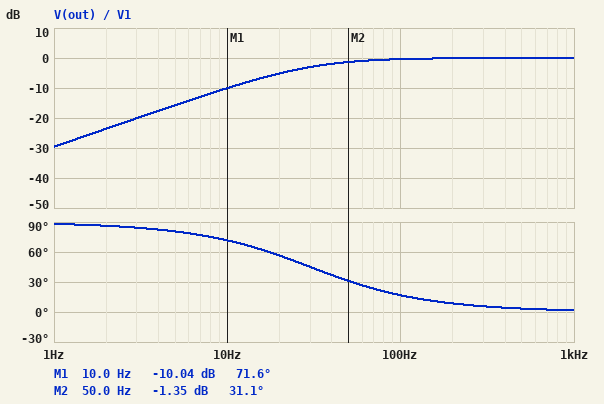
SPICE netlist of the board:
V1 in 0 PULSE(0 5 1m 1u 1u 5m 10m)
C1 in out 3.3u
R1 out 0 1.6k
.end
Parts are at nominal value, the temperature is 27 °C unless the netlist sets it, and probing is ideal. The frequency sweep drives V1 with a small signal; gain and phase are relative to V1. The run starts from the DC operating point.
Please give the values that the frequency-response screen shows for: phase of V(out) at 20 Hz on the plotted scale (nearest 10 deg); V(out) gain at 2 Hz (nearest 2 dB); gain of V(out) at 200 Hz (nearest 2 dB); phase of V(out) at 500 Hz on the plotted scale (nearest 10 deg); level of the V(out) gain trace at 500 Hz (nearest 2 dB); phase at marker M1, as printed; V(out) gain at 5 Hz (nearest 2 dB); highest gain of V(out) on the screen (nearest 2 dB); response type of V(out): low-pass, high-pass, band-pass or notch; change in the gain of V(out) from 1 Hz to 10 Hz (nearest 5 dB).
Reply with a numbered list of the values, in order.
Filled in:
1. 60 deg
2. -24 dB
3. 0 dB
4. 0 deg
5. 0 dB
6. 71.6 deg
7. -16 dB
8. 0 dB
9. high-pass
10. 20 dB
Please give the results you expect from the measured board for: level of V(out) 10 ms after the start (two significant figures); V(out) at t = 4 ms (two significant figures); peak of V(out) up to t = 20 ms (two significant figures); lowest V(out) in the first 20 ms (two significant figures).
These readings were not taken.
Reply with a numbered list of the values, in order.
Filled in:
1. -1.4 V
2. 2.8 V
3. 5.0 V
4. -3.5 V
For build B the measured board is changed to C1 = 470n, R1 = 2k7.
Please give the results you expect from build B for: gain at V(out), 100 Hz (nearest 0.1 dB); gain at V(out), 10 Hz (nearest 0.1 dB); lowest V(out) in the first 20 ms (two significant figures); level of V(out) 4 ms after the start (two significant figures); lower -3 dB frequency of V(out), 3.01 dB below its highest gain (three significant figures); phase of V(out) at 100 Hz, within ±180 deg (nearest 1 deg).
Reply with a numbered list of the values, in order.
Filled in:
1. -4.1 dB
2. -22.0 dB
3. -4.9 V
4. 470 mV
5. 125 Hz
6. 51 deg
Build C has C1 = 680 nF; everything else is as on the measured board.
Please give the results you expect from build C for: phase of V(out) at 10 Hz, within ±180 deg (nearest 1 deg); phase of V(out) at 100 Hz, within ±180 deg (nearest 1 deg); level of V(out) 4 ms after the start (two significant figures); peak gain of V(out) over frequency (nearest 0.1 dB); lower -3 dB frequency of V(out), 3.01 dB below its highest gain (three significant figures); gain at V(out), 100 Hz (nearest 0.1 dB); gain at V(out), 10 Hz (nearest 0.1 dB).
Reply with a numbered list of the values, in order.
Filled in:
1. 86 deg
2. 56 deg
3. 320 mV
4. 0 dB
5. 146 Hz
6. -5.0 dB
7. -23.3 dB
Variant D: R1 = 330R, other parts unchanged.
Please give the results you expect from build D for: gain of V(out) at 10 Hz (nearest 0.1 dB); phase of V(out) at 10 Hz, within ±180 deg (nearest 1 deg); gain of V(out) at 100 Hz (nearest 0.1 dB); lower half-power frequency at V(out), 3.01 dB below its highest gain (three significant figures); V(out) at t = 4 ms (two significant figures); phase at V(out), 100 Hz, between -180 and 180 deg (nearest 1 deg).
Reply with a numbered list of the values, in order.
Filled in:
1. -23.3 dB
2. 86 deg
3. -5.0 dB
4. 146 Hz
5. 320 mV
6. 56 deg
